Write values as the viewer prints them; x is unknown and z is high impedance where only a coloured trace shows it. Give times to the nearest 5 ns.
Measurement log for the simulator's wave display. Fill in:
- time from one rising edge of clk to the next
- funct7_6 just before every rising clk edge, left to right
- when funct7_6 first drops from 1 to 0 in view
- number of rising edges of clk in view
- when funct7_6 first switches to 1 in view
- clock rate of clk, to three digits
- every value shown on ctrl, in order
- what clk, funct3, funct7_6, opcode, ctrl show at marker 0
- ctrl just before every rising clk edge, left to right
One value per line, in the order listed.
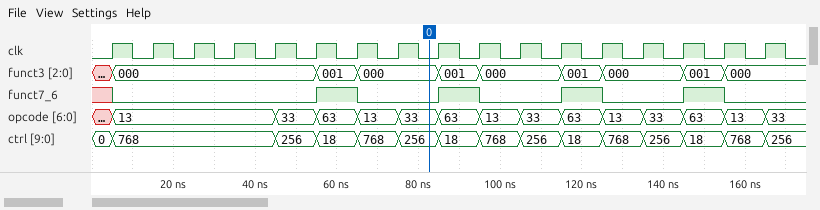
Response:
10 ns
x 0 0 0 0 0 1 0 0 1 0 0 1 0 0 1 0
65 ns
17
55 ns
100 MHz
0, 768, 256, 18, 768, 256, 18, 768, 256, 18, 768, 256, 18, 768, 256
clk=0, funct3=000, funct7_6=0, opcode=33, ctrl=256
0, 768, 768, 768, 768, 256, 18, 768, 256, 18, 768, 256, 18, 768, 256, 18, 768
